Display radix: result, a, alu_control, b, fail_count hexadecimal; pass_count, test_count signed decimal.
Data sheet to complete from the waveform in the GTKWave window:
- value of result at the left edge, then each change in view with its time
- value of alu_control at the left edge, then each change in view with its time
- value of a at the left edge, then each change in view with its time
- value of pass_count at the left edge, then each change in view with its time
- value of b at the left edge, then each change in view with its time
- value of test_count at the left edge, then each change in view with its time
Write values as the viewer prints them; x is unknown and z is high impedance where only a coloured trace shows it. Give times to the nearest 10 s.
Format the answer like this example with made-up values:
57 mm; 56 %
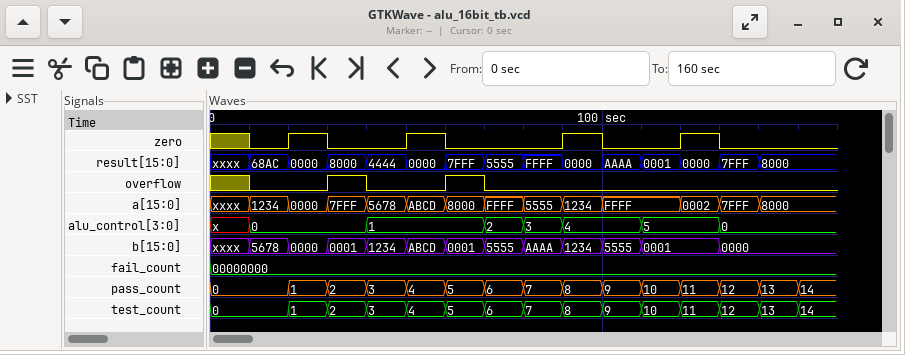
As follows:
xxxx, 68AC at 10 s, 0000 at 20 s, 8000 at 30 s, 4444 at 40 s, 0000 at 50 s, 7FFF at 60 s, 5555 at 70 s, FFFF at 80 s, 0000 at 90 s, AAAA at 100 s, 0001 at 110 s, 0000 at 120 s, 7FFF at 130 s, 8000 at 140 s; x, 0 at 10 s, 1 at 40 s, 2 at 70 s, 3 at 80 s, 4 at 90 s, 5 at 110 s, 0 at 130 s; xxxx, 1234 at 10 s, 0000 at 20 s, 7FFF at 30 s, 5678 at 40 s, ABCD at 50 s, 8000 at 60 s, FFFF at 70 s, 5555 at 80 s, 1234 at 90 s, FFFF at 100 s, 0002 at 120 s, 7FFF at 130 s, 8000 at 140 s; 0, 1 at 20 s, 2 at 30 s, 3 at 40 s, 4 at 50 s, 5 at 60 s, 6 at 70 s, 7 at 80 s, 8 at 90 s, 9 at 100 s, 10 at 110 s, 11 at 120 s, 12 at 130 s, 13 at 140 s, 14 at 150 s; xxxx, 5678 at 10 s, 0000 at 20 s, 0001 at 30 s, 1234 at 40 s, ABCD at 50 s, 0001 at 60 s, 5555 at 70 s, AAAA at 80 s, 1234 at 90 s, 5555 at 100 s, 0001 at 110 s, 0000 at 130 s; 0, 1 at 20 s, 2 at 30 s, 3 at 40 s, 4 at 50 s, 5 at 60 s, 6 at 70 s, 7 at 80 s, 8 at 90 s, 9 at 100 s, 10 at 110 s, 11 at 120 s, 12 at 130 s, 13 at 140 s, 14 at 150 s
